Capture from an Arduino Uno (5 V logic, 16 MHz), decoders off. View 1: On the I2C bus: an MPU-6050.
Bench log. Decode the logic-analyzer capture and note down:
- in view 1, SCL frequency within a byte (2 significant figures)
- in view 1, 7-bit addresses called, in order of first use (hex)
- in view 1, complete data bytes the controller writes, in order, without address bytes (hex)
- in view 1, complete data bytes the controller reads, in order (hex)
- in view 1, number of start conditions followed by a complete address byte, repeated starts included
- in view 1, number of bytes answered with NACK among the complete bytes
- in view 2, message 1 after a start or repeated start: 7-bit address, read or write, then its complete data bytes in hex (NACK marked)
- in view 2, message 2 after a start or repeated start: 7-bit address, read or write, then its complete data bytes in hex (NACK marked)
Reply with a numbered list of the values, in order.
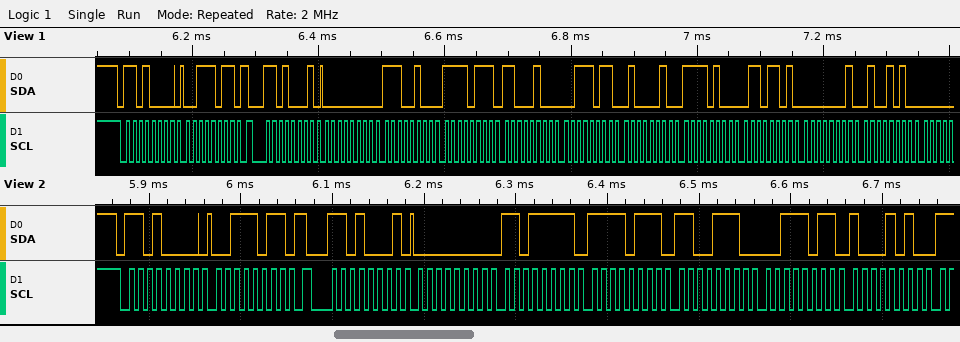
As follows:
1. 100 kHz
2. 0x68
3. 3B
4. 00 E4 F7 C4 3B 42 F4 6D 01 4A
5. 2
6. 0
7. 0x68 write: 3B
8. 0x68 read: 00 DF F7 CE 3B 8A
